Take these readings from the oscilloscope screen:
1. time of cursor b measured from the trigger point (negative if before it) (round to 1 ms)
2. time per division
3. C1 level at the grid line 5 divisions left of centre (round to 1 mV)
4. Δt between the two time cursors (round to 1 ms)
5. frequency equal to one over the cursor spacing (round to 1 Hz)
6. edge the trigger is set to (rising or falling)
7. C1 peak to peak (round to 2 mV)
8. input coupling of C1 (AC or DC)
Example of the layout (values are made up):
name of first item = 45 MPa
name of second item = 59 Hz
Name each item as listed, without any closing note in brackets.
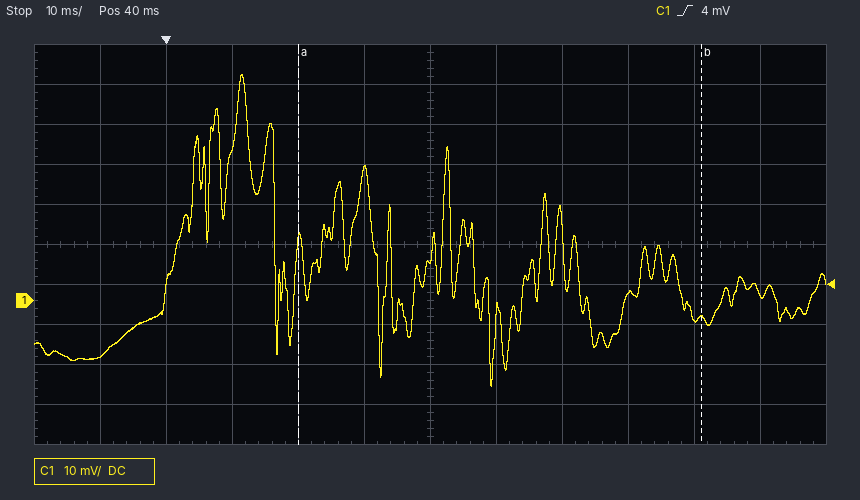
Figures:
time of cursor b measured from the trigger point (negative if before it) = +81 ms
time per division = 10 ms
C1 level at the grid line 5 divisions left of centre = -14 mV
Δt between the two time cursors = 61 ms
frequency equal to one over the cursor spacing = 16 Hz
edge the trigger is set to = rising
C1 peak to peak = 78 mV
input coupling of C1 = DC
